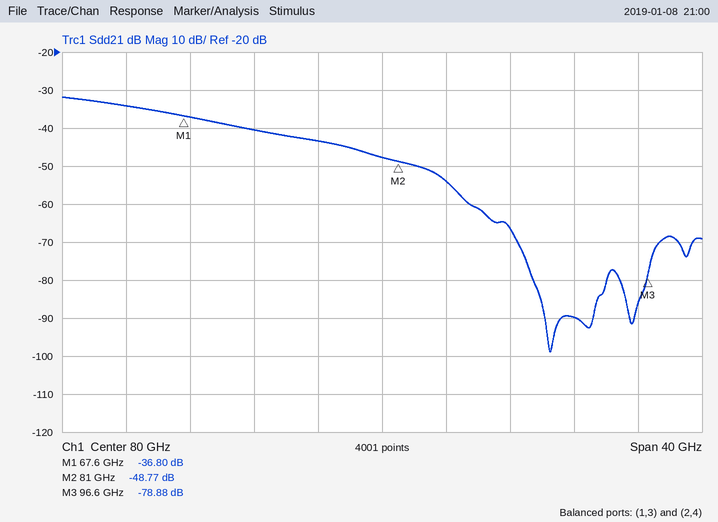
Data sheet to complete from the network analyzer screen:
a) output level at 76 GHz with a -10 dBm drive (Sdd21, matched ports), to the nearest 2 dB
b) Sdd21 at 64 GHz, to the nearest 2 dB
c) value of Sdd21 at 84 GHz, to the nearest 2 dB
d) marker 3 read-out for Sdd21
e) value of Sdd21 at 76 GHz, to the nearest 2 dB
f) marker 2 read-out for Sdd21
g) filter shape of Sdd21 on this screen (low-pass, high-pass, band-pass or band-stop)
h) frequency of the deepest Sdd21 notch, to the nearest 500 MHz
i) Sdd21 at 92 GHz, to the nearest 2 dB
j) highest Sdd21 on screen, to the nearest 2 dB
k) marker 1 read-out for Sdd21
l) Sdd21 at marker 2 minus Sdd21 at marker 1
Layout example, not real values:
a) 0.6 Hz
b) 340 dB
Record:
a) -54 dBm
b) -34 dB
c) -54 dB
d) -78.88 dB
e) -44 dB
f) -48.77 dB
g) low-pass
h) 90.5 GHz
i) -90 dB
j) -32 dB
k) -36.80 dB
l) -11.97 dB
